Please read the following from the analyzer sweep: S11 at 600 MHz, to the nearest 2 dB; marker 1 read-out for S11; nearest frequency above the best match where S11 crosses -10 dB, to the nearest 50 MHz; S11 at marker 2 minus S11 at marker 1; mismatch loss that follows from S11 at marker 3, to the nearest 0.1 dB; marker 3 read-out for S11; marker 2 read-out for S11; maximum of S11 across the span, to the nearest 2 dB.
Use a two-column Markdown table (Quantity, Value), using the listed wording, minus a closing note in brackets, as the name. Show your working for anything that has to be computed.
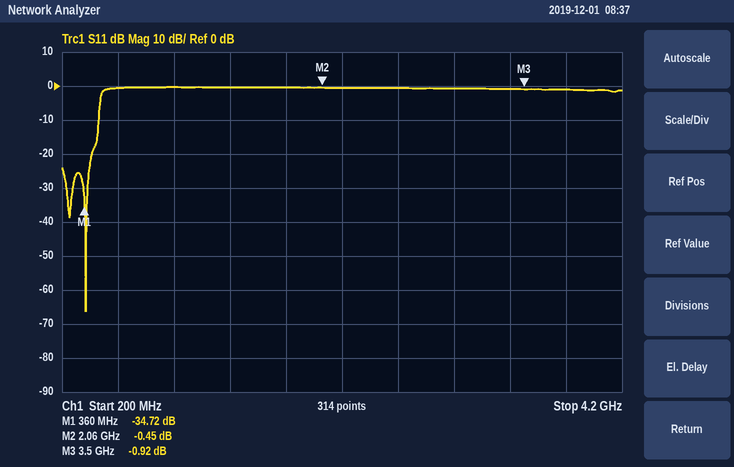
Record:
| Quantity | Value |
|---|---|
| S11 at 600 MHz, to the nearest 2 dB | 0 dB |
| marker 1 read-out for S11 | -34.72 dB |
| nearest frequency above the best match where S11 crosses -10 dB, to the nearest 50 MHz | 450 MHz |
| S11 at marker 2 minus S11 at marker 1 | -0.45 − (-34.72) = 34.27 dB |
| mismatch loss that follows from S11 at marker 3, to the nearest 0.1 dB | −10 log10(1 − 10^(-0.92/10)) ≈ 7.2 dB |
| marker 3 read-out for S11 | -0.92 dB |
| marker 2 read-out for S11 | -0.45 dB |
| maximum of S11 across the span, to the nearest 2 dB | 0 dB |
